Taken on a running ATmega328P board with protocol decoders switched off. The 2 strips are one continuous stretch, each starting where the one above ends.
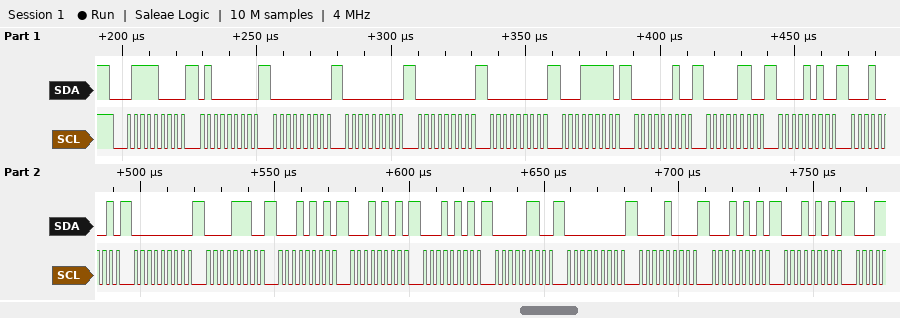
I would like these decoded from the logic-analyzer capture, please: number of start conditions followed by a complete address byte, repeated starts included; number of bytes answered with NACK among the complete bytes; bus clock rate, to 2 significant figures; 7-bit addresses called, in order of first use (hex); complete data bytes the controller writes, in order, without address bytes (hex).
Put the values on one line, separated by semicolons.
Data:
1; 0; 400 kHz; 0x3C; 40 00 00 00 00 1F 02 06 0A 11 00 0E 15 15 15 06 00 08 15 15
